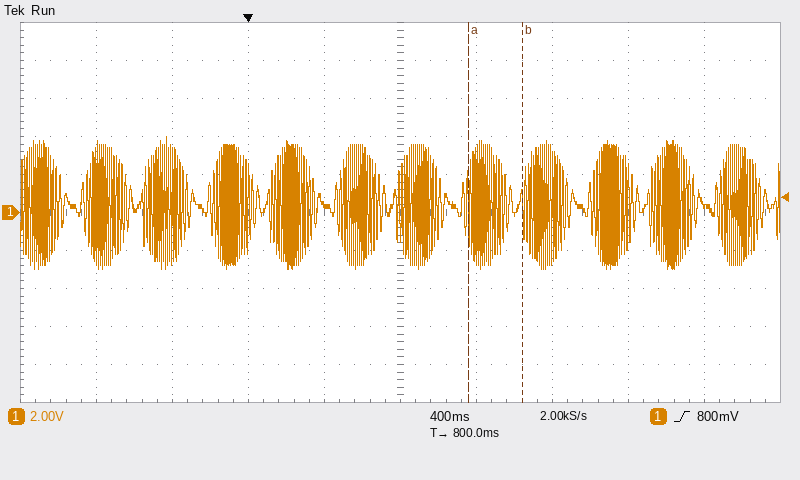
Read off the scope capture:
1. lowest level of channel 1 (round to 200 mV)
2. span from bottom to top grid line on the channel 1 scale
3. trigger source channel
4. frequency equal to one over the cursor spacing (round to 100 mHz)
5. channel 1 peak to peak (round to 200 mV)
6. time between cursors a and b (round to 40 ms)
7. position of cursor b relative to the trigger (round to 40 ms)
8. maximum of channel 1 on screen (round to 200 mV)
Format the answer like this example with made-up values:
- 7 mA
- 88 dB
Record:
- -3.0 V
- 20 V
- channel 1
- 3.6 Hz
- 7.0 V
- 280 ms
- +1.44 s
- 4.0 V
